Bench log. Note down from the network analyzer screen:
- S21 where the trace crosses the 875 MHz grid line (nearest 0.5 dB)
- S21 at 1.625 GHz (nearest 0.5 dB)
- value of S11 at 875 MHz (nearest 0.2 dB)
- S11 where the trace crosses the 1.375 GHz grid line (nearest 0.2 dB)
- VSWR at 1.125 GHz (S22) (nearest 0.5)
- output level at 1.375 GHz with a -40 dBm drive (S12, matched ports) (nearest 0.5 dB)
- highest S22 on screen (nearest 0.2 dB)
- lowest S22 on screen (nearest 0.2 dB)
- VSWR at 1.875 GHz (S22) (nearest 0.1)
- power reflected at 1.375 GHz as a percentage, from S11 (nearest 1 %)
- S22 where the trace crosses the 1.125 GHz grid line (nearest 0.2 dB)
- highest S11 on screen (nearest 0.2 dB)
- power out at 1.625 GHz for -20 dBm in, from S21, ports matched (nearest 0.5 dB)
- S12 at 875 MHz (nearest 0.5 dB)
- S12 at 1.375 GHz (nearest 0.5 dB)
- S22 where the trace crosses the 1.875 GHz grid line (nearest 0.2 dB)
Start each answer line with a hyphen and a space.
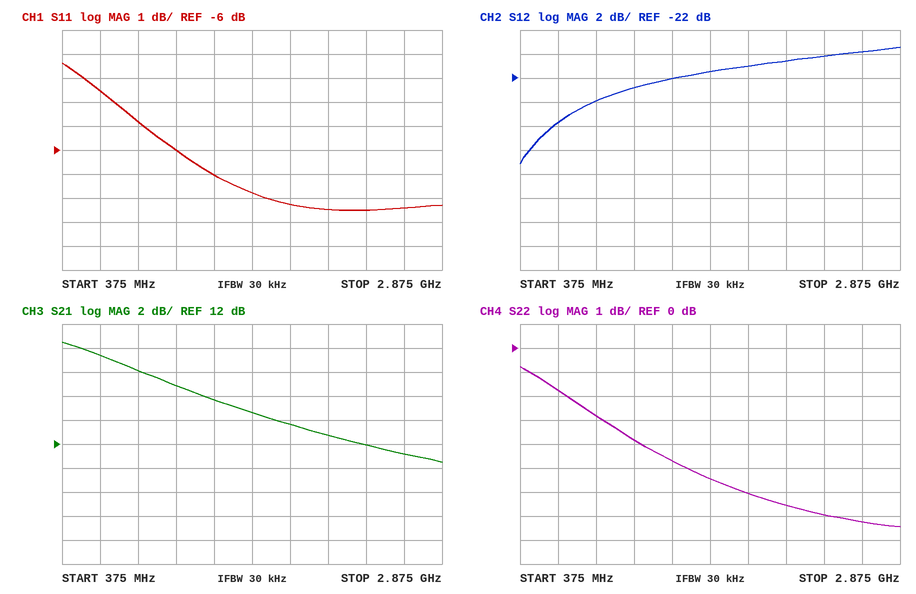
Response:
- 18.0 dB
- 14.5 dB
- -4.8 dB
- -7.0 dB
- 4.5
- -62.0 dBm
- -0.8 dB
- -7.4 dB
- 3.0
- 20 %
- -3.8 dB
- -2.4 dB
- -5.5 dBm
- -24.0 dB
- -22.0 dB
- -6.0 dB
